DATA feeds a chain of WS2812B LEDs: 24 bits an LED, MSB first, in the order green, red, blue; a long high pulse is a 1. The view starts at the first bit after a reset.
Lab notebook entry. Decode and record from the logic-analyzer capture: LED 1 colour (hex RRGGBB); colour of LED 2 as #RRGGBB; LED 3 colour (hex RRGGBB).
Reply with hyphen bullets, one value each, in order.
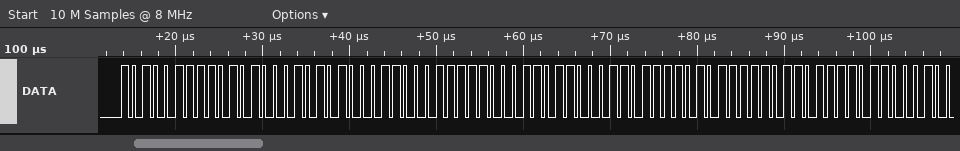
- #A8A7A8
- #C6C7C6
- #F6F5F6
